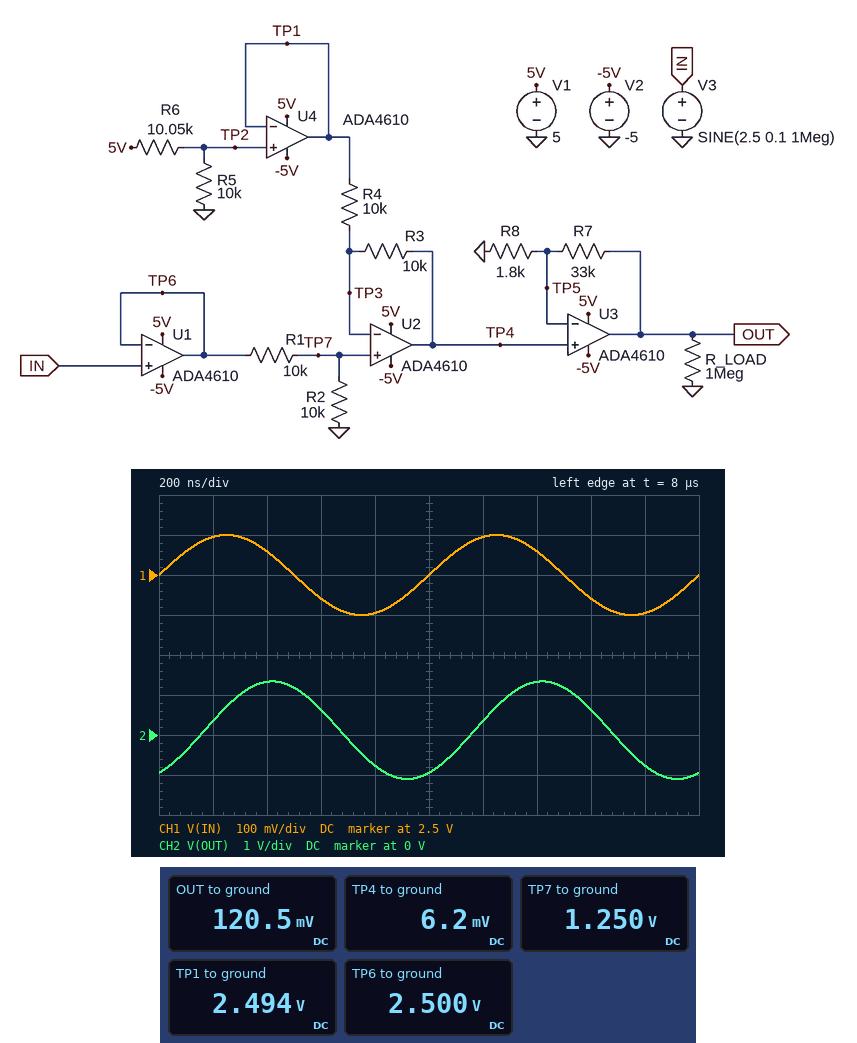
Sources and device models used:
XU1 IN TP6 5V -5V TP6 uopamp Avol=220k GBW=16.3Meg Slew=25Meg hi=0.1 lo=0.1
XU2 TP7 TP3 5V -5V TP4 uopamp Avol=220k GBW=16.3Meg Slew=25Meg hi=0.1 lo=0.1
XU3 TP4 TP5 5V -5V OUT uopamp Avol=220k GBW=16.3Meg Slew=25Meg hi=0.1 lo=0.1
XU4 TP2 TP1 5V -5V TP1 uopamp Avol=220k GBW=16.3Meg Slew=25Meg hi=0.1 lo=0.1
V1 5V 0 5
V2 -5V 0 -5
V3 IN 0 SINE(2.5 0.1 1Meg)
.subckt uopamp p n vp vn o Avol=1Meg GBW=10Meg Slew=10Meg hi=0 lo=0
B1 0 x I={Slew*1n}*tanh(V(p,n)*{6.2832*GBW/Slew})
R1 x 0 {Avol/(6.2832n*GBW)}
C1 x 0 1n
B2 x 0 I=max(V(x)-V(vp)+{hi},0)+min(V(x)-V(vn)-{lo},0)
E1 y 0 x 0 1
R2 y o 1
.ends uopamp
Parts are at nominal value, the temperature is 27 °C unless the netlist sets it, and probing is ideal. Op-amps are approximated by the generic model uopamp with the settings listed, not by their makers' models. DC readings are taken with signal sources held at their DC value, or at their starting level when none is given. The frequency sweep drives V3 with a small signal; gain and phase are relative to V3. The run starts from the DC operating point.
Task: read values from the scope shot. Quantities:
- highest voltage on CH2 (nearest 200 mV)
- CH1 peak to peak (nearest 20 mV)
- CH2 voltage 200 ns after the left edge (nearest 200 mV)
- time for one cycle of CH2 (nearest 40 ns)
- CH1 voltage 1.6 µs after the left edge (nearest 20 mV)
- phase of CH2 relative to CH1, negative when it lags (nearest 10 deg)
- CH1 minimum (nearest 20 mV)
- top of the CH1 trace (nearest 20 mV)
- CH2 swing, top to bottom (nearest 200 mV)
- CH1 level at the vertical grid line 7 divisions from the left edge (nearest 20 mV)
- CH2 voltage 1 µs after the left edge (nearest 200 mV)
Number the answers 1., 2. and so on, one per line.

1. 1.4 V
2. 200 mV
3. 400 mV
4. 1.00 µs
5. 2.44 V
6. -60 deg
7. 2.40 V
8. 2.60 V
9. 2.4 V
10. 2.56 V
11. -1.0 V
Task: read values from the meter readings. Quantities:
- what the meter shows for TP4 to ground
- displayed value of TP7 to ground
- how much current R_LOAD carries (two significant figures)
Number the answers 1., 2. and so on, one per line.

1. 6.2 mV
2. 1.250 V
3. 120 nA
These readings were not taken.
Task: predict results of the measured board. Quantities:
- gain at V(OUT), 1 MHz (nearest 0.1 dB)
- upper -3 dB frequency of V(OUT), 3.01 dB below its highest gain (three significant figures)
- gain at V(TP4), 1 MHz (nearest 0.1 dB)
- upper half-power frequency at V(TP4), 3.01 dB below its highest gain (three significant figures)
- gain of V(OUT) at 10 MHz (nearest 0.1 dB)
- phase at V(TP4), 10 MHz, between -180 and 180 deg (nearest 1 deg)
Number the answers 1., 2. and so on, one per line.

1. 21.8 dB
2. 832 kHz
3. -0.1 dB
4. 6.83 MHz
5. -1.2 dB
6. -82 deg
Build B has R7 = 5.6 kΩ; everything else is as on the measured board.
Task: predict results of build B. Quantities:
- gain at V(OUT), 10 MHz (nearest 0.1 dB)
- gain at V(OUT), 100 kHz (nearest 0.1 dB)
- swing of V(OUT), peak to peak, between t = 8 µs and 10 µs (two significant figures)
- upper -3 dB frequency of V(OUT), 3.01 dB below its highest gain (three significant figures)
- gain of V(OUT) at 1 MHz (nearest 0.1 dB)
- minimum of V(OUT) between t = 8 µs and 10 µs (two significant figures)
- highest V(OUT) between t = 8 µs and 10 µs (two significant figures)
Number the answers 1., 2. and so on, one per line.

1. -1.8 dB
2. 12.3 dB
3. 790 mV
4. 3.23 MHz
5. 11.9 dB
6. -370 mV
7. 420 mV
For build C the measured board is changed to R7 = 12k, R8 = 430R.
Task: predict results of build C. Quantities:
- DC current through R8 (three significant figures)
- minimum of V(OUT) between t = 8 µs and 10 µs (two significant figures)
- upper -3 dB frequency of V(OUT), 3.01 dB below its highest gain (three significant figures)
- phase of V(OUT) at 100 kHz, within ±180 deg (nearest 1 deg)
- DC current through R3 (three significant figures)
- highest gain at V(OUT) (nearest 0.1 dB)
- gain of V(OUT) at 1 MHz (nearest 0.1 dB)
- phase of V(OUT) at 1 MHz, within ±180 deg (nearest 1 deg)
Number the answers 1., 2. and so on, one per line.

1. 14.5 µA
2. -1.2 V
3. 561 kHz
4. -11 deg
5. 124 µA
6. 29.2 dB
7. 23.0 dB
8. -71 deg
